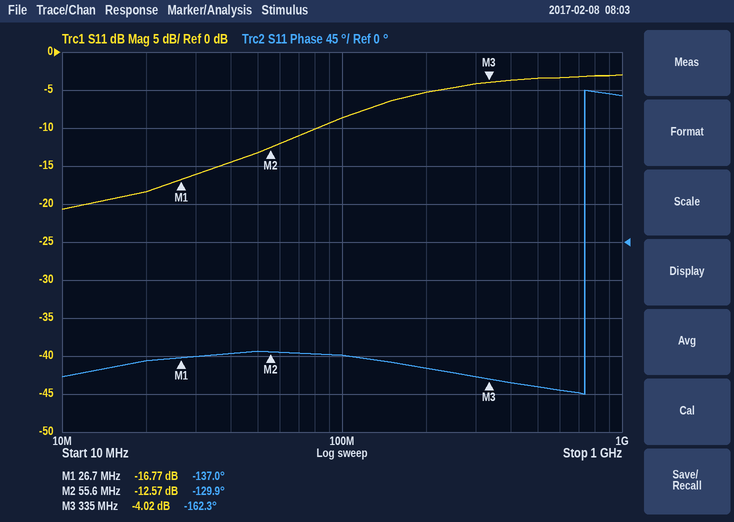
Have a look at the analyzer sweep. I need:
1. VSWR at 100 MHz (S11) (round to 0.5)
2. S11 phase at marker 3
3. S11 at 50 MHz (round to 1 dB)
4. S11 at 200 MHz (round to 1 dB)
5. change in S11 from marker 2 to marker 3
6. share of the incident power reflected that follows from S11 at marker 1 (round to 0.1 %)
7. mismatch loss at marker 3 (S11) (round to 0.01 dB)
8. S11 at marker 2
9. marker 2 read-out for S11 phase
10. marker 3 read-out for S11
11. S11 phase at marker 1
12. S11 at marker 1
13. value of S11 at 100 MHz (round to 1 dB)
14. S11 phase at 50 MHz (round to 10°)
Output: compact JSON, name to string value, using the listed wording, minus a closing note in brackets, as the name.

{"VSWR at 100 MHz (S11)": "2.0", "S11 phase at marker 3": "-162.3°", "S11 at 50 MHz": "-13 dB", "S11 at 200 MHz": "-5 dB", "change in S11 from marker 2 to marker 3": "8.55 dB", "share of the incident power reflected that follows from S11 at marker 1": "2.1 %", "mismatch loss at marker 3 (S11)": "2.19 dB", "S11 at marker 2": "-12.57 dB", "marker 2 read-out for S11 phase": "-129.9°", "marker 3 read-out for S11": "-4.02 dB", "S11 phase at marker 1": "-137.0°", "S11 at marker 1": "-16.77 dB", "value of S11 at 100 MHz": "-9 dB", "S11 phase at 50 MHz": "-130°"}
